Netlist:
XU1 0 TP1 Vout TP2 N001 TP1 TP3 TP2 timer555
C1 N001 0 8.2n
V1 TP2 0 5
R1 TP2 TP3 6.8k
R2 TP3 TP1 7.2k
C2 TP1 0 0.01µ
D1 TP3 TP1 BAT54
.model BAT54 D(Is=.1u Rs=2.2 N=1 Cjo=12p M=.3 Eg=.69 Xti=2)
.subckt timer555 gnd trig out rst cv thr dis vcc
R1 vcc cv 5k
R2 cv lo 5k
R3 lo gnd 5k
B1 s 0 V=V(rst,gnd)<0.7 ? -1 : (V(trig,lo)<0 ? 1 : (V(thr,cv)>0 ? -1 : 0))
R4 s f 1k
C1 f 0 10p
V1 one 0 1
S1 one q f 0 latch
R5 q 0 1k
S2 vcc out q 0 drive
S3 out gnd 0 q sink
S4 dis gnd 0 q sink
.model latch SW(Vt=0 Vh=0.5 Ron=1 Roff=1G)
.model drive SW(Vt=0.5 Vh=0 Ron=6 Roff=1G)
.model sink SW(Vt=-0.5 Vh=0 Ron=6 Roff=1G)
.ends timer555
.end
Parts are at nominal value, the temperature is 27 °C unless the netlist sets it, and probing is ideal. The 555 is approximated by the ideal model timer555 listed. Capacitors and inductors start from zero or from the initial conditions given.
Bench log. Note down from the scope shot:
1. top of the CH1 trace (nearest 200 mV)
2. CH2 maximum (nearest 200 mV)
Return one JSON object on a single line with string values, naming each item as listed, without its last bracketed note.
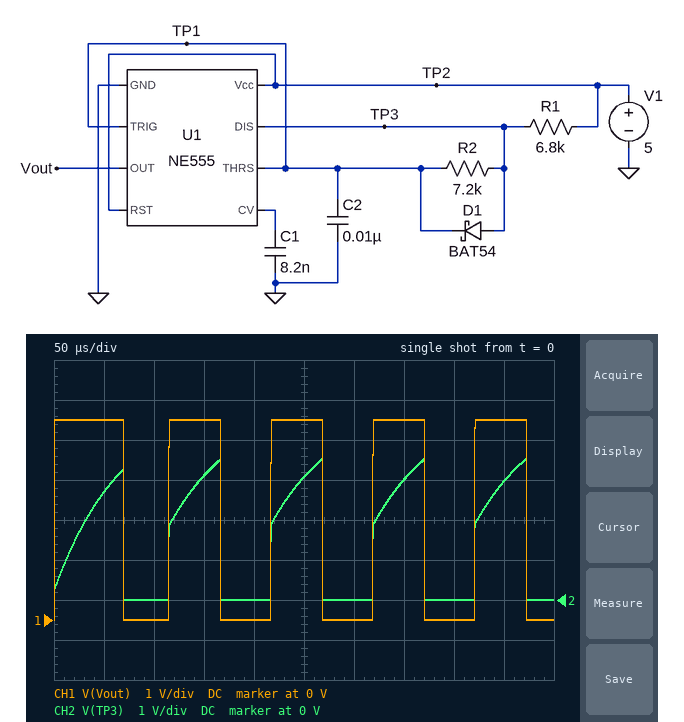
{"top of the CH1 trace": "5.0 V", "CH2 maximum": "3.6 V"}
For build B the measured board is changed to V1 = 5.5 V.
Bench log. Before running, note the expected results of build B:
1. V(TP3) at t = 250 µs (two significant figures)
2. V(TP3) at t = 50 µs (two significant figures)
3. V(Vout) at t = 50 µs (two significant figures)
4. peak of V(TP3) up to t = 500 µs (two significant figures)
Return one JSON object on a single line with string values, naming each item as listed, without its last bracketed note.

{"V(TP3) at t = 250 µs": "3.4 V", "V(TP3) at t = 50 µs": "3.0 V", "V(Vout) at t = 50 µs": "5.5 V", "peak of V(TP3) up to t = 500 µs": "3.9 V"}
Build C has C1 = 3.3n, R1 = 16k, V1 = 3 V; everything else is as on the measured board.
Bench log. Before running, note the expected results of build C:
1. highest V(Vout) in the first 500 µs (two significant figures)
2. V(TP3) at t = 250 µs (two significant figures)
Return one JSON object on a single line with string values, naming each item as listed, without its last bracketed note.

{"highest V(Vout) in the first 500 µs": "3.0 V", "V(TP3) at t = 250 µs": "1.2 V"}
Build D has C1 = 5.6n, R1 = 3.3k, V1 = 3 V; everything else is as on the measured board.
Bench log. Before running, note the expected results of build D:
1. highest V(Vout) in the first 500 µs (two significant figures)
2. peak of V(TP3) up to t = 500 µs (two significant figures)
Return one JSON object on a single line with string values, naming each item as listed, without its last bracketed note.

{"highest V(Vout) in the first 500 µs": "3.0 V", "peak of V(TP3) up to t = 500 µs": "2.2 V"}
